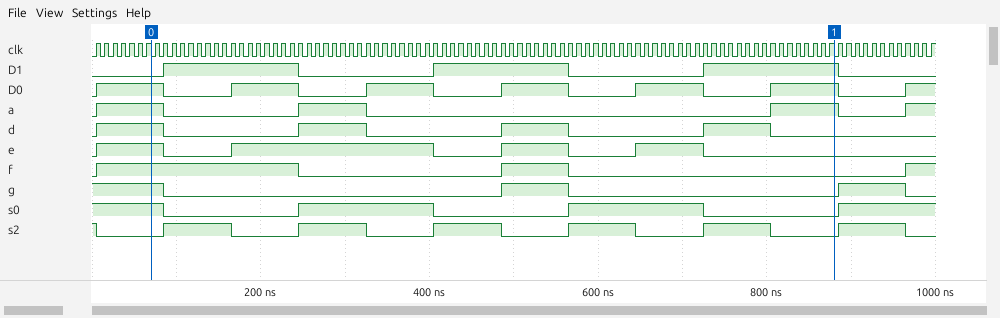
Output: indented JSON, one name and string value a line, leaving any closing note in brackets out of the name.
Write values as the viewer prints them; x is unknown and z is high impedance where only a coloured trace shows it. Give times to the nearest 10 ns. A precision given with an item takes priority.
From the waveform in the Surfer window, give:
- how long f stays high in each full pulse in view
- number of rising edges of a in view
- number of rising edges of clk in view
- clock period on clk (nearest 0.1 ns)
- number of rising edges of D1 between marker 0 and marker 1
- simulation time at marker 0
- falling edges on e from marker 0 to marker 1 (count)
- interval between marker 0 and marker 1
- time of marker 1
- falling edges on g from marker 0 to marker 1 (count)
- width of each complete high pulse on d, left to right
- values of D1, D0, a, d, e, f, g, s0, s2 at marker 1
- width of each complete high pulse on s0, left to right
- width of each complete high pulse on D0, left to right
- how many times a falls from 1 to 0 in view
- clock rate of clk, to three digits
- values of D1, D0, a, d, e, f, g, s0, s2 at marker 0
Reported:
{
  "how long f stays high in each full pulse in view": "240 ns, 80 ns",
  "number of rising edges of a in view": "4",
  "number of rising edges of clk in view": "100",
  "clock period on clk": "10 ns",
  "number of rising edges of D1 between marker 0 and marker 1": "3",
  "simulation time at marker 0": "70 ns",
  "falling edges on e from marker 0 to marker 1": "4",
  "interval between marker 0 and marker 1": "810 ns",
  "time of marker 1": "880 ns",
  "falling edges on g from marker 0 to marker 1": "2",
  "width of each complete high pulse on d, left to right": "80 ns, 80 ns, 80 ns, 80 ns",
  "values of D1, D0, a, d, e, f, g, s0, s2 at marker 1": "D1=1, D0=1, a=1, d=0, e=0, f=0, g=0, s0=0, s2=0",
  "width of each complete high pulse on s0, left to right": "160 ns, 160 ns",
  "width of each complete high pulse on D0, left to right": "80 ns, 80 ns, 80 ns, 80 ns, 80 ns, 80 ns",
  "how many times a falls from 1 to 0 in view": "3",
  "clock rate of clk, to three digits": "100 MHz",
  "values of D1, D0, a, d, e, f, g, s0, s2 at marker 0": "D1=0, D0=1, a=1, d=1, e=1, f=1, g=1, s0=1, s2=0"
}
